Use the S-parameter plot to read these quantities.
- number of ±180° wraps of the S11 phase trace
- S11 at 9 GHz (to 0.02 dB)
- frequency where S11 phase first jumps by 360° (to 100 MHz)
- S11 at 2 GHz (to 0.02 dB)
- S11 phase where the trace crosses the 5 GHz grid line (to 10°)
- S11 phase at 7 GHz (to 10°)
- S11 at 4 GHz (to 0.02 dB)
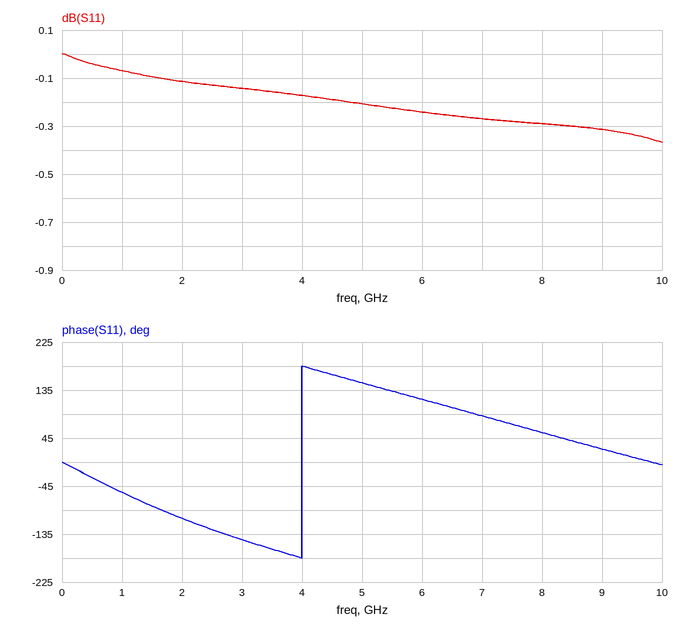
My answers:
1
-0.32 dB
4.0 GHz
-0.12 dB
150°
90°
-0.18 dB
